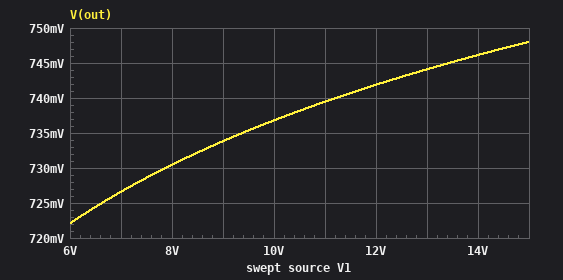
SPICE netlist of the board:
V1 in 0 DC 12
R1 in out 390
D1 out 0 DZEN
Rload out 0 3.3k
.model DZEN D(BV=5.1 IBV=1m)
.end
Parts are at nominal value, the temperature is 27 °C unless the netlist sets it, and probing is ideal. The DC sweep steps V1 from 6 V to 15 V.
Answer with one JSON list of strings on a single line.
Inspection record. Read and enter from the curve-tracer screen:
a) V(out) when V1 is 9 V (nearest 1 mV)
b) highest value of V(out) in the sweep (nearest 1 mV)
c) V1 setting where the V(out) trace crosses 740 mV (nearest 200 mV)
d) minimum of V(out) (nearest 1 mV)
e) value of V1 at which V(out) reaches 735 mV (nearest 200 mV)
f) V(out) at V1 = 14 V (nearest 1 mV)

["734 mV", "748 mV", "11.2 V", "722 mV", "9.4 V", "746 mV"]
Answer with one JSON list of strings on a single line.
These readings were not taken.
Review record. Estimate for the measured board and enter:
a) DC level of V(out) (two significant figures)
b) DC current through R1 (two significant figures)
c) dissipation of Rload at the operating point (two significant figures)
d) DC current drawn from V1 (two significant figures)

["740 mV", "29 mA", "170 µW", "29 mA"]
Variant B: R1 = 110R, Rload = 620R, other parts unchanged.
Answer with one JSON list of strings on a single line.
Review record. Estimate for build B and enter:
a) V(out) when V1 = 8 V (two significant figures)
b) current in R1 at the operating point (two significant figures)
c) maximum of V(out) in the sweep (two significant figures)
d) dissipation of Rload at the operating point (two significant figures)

["760 mV", "100 mA", "780 mV", "970 µW"]
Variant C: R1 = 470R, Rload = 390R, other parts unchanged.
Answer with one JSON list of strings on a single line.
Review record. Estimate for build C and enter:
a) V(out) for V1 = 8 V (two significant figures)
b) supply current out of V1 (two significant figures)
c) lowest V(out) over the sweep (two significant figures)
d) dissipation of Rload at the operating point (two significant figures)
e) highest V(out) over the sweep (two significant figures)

["720 mV", "24 mA", "710 mV", "1.4 mW", "740 mV"]
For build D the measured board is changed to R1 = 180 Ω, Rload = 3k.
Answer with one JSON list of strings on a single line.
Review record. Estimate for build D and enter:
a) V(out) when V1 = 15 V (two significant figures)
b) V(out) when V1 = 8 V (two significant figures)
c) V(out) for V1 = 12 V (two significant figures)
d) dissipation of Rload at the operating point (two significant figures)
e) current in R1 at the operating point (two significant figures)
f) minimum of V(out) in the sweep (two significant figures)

["770 mV", "750 mV", "760 mV", "190 µW", "62 mA", "740 mV"]
